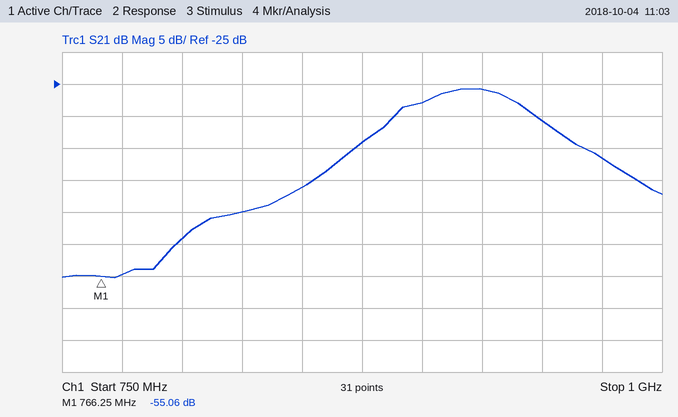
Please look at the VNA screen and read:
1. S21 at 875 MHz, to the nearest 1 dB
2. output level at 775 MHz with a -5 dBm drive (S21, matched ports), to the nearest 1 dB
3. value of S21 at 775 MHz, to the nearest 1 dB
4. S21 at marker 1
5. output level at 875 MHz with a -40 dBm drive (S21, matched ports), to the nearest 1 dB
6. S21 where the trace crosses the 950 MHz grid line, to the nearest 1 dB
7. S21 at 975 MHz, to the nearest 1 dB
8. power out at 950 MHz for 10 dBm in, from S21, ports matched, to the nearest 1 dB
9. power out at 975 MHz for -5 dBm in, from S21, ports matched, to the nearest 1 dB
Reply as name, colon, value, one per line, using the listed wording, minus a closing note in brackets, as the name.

S21 at 875 MHz, to the nearest 1 dB: -34 dB
output level at 775 MHz with a -5 dBm drive (S21, matched ports), to the nearest 1 dB: -60 dBm
value of S21 at 775 MHz, to the nearest 1 dB: -55 dB
S21 at marker 1: -55.06 dB
output level at 875 MHz with a -40 dBm drive (S21, matched ports), to the nearest 1 dB: -74 dBm
S21 where the trace crosses the 950 MHz grid line, to the nearest 1 dB: -31 dB
S21 at 975 MHz, to the nearest 1 dB: -37 dB
power out at 950 MHz for 10 dBm in, from S21, ports matched, to the nearest 1 dB: -21 dBm
power out at 975 MHz for -5 dBm in, from S21, ports matched, to the nearest 1 dB: -42 dBm
